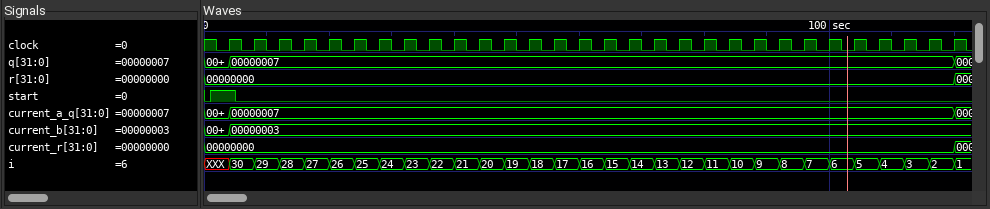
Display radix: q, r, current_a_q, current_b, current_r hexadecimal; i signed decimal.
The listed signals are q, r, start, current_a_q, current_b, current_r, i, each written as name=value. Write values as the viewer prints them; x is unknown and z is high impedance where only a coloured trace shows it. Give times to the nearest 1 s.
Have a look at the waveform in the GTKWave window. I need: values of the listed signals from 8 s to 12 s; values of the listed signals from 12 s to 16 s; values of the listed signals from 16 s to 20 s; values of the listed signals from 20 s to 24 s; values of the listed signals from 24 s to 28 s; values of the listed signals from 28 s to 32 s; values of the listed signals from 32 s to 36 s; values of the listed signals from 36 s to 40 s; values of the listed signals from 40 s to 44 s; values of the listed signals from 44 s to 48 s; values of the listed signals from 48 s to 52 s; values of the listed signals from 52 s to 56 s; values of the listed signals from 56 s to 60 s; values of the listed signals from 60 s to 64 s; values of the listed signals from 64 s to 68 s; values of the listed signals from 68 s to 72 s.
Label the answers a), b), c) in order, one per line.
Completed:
a) q=00000007, r=00000000, start=0, current_a_q=00000007, current_b=00000003, current_r=00000000, i=29
b) q=00000007, r=00000000, start=0, current_a_q=00000007, current_b=00000003, current_r=00000000, i=28
c) q=00000007, r=00000000, start=0, current_a_q=00000007, current_b=00000003, current_r=00000000, i=27
d) q=00000007, r=00000000, start=0, current_a_q=00000007, current_b=00000003, current_r=00000000, i=26
e) q=00000007, r=00000000, start=0, current_a_q=00000007, current_b=00000003, current_r=00000000, i=25
f) q=00000007, r=00000000, start=0, current_a_q=00000007, current_b=00000003, current_r=00000000, i=24
g) q=00000007, r=00000000, start=0, current_a_q=00000007, current_b=00000003, current_r=00000000, i=23
h) q=00000007, r=00000000, start=0, current_a_q=00000007, current_b=00000003, current_r=00000000, i=22
i) q=00000007, r=00000000, start=0, current_a_q=00000007, current_b=00000003, current_r=00000000, i=21
j) q=00000007, r=00000000, start=0, current_a_q=00000007, current_b=00000003, current_r=00000000, i=20
k) q=00000007, r=00000000, start=0, current_a_q=00000007, current_b=00000003, current_r=00000000, i=19
l) q=00000007, r=00000000, start=0, current_a_q=00000007, current_b=00000003, current_r=00000000, i=18
m) q=00000007, r=00000000, start=0, current_a_q=00000007, current_b=00000003, current_r=00000000, i=17
n) q=00000007, r=00000000, start=0, current_a_q=00000007, current_b=00000003, current_r=00000000, i=16
o) q=00000007, r=00000000, start=0, current_a_q=00000007, current_b=00000003, current_r=00000000, i=15
p) q=00000007, r=00000000, start=0, current_a_q=00000007, current_b=00000003, current_r=00000000, i=14
